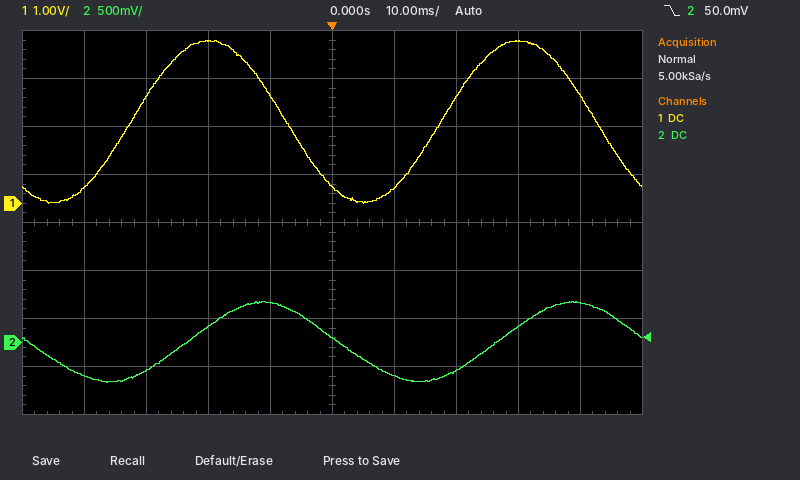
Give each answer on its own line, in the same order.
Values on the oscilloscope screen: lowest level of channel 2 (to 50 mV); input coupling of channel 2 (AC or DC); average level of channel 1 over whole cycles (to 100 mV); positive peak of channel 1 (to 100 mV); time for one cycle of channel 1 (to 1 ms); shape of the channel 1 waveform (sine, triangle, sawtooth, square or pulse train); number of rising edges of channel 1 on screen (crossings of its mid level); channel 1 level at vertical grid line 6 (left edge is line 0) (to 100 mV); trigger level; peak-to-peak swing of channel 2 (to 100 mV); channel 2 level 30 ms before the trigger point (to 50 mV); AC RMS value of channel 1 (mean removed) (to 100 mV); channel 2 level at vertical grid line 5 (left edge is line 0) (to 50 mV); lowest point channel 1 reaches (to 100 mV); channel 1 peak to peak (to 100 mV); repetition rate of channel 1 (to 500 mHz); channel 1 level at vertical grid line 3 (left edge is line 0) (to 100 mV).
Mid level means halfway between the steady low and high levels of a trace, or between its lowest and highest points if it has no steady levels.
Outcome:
-400 mV
DC
1.7 V
3.4 V
50 ms
sine
2
300 mV
50.0 mV
800 mV
-300 mV
1.2 V
50 mV
0.0 V
3.4 V
20.0 Hz
3.4 V
